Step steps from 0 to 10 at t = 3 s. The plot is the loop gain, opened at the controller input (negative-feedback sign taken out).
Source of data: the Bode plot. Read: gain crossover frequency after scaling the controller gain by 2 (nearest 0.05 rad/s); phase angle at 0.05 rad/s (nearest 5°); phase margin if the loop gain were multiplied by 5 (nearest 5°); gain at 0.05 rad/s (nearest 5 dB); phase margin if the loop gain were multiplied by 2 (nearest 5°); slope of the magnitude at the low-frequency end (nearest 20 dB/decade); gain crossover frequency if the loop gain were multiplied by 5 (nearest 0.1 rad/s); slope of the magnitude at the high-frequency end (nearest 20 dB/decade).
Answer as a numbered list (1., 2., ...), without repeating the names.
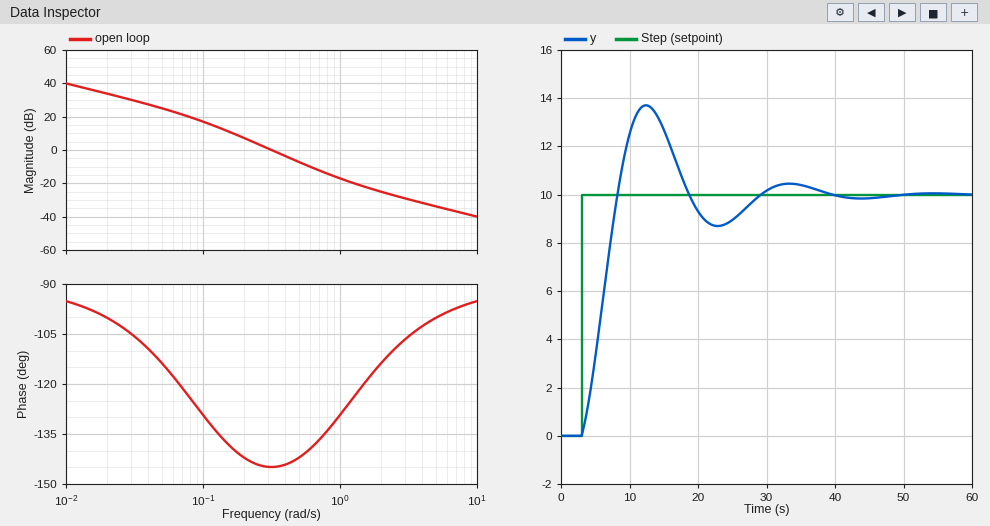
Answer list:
1. 0.45 rad/s
2. -115°
3. 45°
4. 25 dB
5. 35°
6. -20 dB/decade
7. 0.8 rad/s
8. -20 dB/decade
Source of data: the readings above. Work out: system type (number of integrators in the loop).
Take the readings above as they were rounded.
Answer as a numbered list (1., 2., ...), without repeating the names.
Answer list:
1. 1
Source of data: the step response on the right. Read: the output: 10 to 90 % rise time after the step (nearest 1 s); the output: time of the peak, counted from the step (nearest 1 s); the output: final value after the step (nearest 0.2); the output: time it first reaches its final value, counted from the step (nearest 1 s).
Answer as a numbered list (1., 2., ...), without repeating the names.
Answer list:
1. 4 s
2. 9 s
3. 10.0
4. 5 s
